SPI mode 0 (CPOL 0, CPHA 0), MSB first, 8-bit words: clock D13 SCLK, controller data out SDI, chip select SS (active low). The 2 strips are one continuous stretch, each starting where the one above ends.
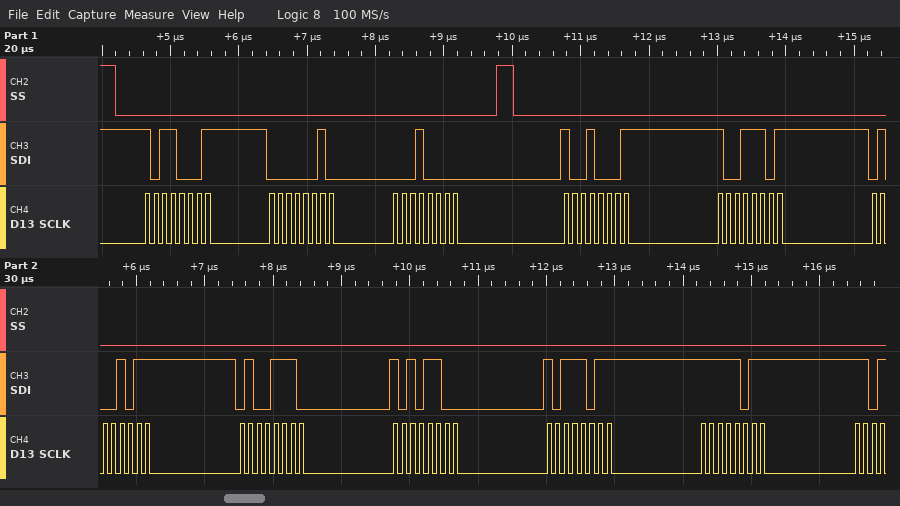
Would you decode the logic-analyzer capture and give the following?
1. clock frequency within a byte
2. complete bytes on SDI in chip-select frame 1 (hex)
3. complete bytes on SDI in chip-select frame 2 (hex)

8 MHz
B1 02 10
91 9D 4B 4E AC BB FB
